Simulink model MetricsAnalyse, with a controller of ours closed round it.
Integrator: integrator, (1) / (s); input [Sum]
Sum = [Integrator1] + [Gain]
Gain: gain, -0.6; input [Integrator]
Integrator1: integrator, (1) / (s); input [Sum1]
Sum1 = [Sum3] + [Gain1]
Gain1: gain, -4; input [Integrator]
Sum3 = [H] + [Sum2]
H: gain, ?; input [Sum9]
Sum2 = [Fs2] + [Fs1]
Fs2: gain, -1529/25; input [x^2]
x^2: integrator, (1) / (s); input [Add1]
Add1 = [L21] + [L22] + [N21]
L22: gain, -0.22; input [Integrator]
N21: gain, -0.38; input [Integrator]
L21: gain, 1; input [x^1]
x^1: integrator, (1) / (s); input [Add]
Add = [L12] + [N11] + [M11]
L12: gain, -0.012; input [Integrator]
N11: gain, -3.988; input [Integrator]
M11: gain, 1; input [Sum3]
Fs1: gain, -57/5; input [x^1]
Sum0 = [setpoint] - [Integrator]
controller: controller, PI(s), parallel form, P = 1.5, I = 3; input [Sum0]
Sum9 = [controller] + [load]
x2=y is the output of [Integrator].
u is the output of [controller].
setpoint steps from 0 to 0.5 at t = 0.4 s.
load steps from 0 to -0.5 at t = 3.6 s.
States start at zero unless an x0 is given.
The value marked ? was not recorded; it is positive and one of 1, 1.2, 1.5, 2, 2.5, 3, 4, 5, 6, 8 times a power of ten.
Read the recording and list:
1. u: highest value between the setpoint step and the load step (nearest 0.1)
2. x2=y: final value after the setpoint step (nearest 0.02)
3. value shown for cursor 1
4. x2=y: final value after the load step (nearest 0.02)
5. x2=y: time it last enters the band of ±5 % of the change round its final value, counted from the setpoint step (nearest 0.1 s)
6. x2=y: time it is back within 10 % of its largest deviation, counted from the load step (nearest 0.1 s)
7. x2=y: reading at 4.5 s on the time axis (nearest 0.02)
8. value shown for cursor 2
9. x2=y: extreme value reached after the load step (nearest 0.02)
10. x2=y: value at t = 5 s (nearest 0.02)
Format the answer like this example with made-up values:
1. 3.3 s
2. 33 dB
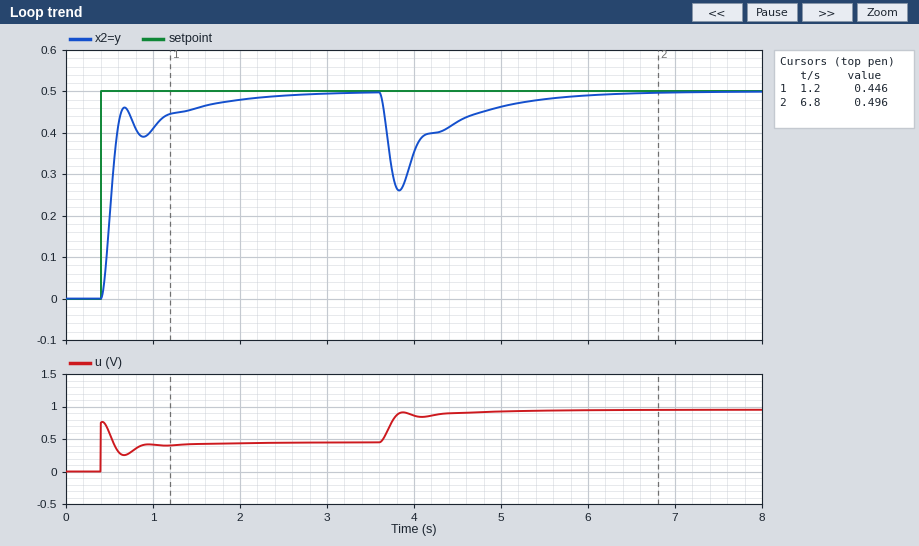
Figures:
1. 0.8
2. 0.50
3. 0.446
4. 0.50
5. 1.4 s
6. 1.7 s
7. 0.42
8. 0.496
9. 0.26
10. 0.46
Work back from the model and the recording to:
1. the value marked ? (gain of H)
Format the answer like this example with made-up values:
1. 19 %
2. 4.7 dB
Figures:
1. 80
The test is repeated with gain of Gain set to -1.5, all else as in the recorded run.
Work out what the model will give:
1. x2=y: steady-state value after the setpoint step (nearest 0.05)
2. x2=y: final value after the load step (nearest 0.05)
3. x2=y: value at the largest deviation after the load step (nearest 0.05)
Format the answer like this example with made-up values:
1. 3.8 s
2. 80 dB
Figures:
1. 0.40
2. 0.40
3. 0.20
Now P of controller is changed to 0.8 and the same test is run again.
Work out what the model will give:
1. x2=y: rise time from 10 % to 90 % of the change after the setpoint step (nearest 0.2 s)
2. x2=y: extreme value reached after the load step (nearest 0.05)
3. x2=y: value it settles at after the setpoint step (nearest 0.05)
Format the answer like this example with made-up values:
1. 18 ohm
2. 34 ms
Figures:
1. 0.8 s
2. 0.20
3. 0.50
